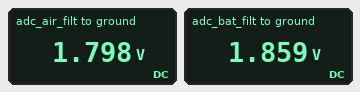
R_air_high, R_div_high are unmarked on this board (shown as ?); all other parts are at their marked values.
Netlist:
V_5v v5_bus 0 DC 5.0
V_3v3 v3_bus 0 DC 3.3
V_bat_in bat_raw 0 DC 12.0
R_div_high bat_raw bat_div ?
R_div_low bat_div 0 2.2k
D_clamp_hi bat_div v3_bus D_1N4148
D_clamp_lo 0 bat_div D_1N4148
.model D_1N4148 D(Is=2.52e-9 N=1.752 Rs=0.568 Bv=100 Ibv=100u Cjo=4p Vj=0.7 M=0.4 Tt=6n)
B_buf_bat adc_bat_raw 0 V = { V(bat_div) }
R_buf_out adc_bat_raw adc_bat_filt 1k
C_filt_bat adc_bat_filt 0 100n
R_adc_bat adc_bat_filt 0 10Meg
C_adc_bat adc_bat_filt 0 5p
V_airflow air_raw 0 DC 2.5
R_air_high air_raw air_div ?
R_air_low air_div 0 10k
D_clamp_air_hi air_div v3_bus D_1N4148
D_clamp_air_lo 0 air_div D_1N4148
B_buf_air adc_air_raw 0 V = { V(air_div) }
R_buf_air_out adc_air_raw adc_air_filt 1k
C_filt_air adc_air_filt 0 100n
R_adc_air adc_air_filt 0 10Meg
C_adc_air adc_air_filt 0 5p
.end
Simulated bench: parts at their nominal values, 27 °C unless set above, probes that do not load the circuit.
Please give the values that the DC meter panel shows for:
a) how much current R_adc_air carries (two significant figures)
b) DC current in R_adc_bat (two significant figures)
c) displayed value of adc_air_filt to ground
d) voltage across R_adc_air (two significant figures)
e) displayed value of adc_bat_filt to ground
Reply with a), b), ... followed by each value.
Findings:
a) 180 nA
b) 190 nA
c) 1.798 V
d) 1.8 V
e) 1.859 V
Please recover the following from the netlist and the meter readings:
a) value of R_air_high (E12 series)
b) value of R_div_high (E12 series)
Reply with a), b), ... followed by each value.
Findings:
a) 3.9 kΩ
b) 12 kΩ
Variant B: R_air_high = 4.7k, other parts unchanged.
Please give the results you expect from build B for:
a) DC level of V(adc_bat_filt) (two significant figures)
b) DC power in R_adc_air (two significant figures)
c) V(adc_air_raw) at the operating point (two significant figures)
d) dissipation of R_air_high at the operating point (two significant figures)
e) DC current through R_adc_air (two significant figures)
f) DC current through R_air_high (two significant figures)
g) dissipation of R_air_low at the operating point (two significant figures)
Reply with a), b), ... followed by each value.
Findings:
a) 1.9 V
b) 290 nW
c) 1.7 V
d) 140 µW
e) 170 nA
f) 170 µA
g) 290 µW
